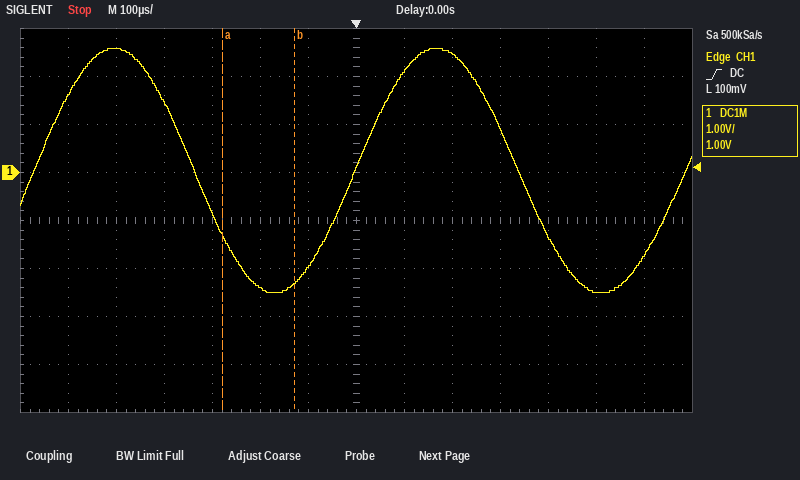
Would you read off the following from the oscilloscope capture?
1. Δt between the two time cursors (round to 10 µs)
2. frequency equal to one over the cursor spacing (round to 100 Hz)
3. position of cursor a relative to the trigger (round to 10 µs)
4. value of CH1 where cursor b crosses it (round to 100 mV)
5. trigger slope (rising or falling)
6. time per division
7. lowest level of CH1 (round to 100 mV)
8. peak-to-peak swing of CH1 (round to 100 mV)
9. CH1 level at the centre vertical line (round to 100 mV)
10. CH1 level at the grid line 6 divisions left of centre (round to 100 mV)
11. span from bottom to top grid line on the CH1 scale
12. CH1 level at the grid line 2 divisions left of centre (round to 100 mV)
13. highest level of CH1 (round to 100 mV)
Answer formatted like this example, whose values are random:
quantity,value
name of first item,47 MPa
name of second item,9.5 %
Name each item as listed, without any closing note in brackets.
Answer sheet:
quantity,value
Δt between the two time cursors,150 µs
frequency equal to one over the cursor spacing,6.7 kHz
position of cursor a relative to the trigger,-280 µs
value of CH1 where cursor b crosses it,-2.3 V
trigger slope,rising
time per division,100 µs
lowest level of CH1,-2.5 V
peak-to-peak swing of CH1,5.1 V
CH1 level at the centre vertical line,100 mV
CH1 level at the grid line 6 divisions left of centre,1.6 V
span from bottom to top grid line on the CH1 scale,8 V
CH1 level at the grid line 2 divisions left of centre,-2.4 V
highest level of CH1,2.6 V
